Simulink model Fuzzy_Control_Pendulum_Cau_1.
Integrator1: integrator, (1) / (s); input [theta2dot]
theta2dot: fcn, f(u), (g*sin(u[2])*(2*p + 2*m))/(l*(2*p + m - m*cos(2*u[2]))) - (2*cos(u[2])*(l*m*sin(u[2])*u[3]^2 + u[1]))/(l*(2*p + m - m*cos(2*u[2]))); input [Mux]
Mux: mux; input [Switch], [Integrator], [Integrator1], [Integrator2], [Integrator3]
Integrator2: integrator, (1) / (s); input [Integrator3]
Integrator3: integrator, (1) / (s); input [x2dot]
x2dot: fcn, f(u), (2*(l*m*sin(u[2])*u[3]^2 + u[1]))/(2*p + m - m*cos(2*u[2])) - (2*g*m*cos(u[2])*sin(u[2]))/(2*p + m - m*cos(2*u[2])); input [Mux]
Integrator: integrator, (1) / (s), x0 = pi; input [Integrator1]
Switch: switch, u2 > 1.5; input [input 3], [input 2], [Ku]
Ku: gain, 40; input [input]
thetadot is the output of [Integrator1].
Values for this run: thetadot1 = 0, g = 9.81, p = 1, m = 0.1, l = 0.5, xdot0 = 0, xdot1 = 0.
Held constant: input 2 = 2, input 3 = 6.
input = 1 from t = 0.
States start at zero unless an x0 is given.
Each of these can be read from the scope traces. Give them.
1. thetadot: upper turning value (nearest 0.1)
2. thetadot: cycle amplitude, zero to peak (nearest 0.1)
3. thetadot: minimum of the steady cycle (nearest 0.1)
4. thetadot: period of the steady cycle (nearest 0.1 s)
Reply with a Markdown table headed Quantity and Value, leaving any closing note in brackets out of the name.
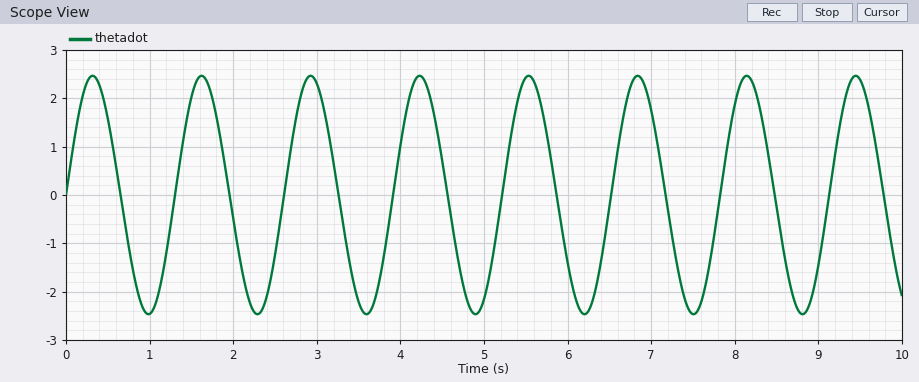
| Quantity | Value |
|---|---|
| thetadot: upper turning value | 2.5 |
| thetadot: cycle amplitude, zero to peak | 2.5 |
| thetadot: minimum of the steady cycle | -2.5 |
| thetadot: period of the steady cycle | 1.3 s |
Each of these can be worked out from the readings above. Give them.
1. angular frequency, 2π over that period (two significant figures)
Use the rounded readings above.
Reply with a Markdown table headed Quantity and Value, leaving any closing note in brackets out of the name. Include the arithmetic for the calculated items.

| Quantity | Value |
|---|---|
| angular frequency, 2π over that period | 2π / 1.3 = 4.8 rad/s |
